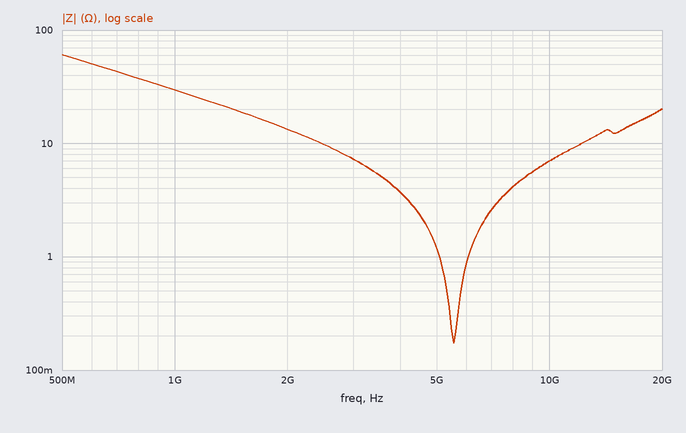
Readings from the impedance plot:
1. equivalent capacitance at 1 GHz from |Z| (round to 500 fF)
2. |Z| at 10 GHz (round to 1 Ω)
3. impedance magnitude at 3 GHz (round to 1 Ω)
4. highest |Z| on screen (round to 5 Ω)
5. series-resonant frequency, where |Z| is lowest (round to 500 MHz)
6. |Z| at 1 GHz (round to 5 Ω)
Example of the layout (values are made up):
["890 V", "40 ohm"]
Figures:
["5.5 pF", "7 Ω", "7 Ω", "60 Ω", "5.5 GHz", "30 Ω"]
